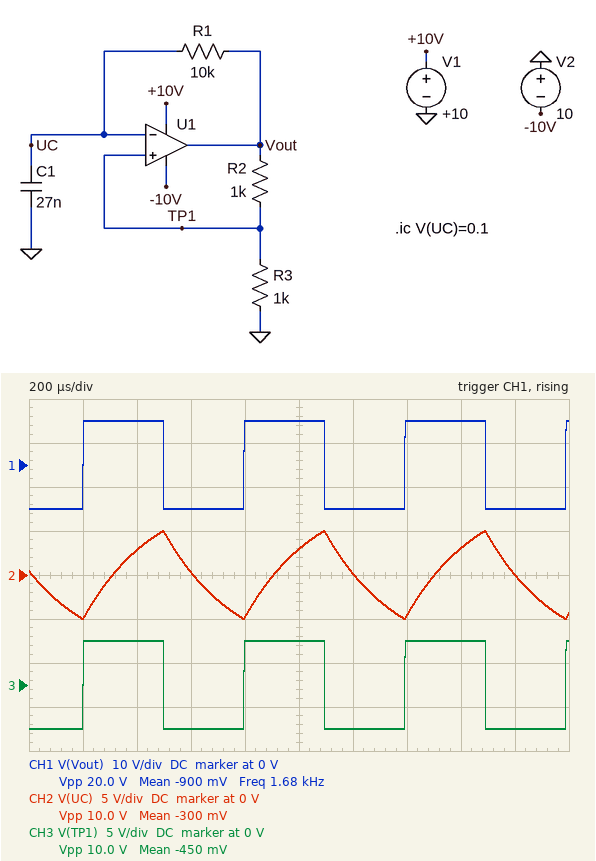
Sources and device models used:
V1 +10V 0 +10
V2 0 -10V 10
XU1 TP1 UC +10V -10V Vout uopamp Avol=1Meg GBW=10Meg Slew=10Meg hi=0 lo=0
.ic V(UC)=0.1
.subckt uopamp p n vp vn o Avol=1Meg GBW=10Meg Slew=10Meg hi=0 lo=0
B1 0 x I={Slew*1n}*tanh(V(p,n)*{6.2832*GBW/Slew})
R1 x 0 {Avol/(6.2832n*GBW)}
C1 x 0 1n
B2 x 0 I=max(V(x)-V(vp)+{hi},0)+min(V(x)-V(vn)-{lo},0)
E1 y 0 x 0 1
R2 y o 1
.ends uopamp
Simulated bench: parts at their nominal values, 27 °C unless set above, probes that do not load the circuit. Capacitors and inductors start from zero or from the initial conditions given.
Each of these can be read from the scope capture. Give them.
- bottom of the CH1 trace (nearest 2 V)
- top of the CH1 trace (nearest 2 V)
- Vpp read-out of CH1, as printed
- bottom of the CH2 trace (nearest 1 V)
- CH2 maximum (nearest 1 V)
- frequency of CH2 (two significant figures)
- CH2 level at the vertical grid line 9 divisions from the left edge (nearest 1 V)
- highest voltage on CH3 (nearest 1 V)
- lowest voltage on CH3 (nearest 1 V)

-10 V
10 V
20.0 V
-5 V
5 V
1.7 kHz
0 V
5 V
-5 V
